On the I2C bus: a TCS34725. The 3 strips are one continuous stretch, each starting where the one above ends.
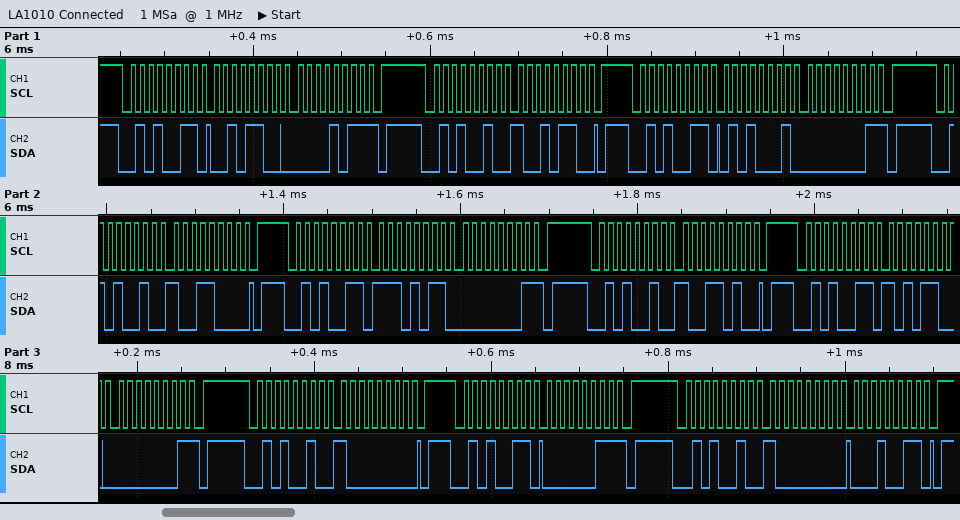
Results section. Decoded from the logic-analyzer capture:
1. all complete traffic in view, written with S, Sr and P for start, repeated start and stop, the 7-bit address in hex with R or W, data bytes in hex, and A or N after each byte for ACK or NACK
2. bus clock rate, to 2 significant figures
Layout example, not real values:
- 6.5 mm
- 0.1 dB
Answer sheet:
- S 29R A 2C A 0B N P S 29W A 96 A P S 29R A 51 A 01 N P S 29W A 98 A P S 29R A EB A 01 N P S 29W A 9A A P S 29R A AC A 01 N P S 29W A 80 A P S 29R A 03 N P S 29W A 80 A 13 A P
- 100 kHz
